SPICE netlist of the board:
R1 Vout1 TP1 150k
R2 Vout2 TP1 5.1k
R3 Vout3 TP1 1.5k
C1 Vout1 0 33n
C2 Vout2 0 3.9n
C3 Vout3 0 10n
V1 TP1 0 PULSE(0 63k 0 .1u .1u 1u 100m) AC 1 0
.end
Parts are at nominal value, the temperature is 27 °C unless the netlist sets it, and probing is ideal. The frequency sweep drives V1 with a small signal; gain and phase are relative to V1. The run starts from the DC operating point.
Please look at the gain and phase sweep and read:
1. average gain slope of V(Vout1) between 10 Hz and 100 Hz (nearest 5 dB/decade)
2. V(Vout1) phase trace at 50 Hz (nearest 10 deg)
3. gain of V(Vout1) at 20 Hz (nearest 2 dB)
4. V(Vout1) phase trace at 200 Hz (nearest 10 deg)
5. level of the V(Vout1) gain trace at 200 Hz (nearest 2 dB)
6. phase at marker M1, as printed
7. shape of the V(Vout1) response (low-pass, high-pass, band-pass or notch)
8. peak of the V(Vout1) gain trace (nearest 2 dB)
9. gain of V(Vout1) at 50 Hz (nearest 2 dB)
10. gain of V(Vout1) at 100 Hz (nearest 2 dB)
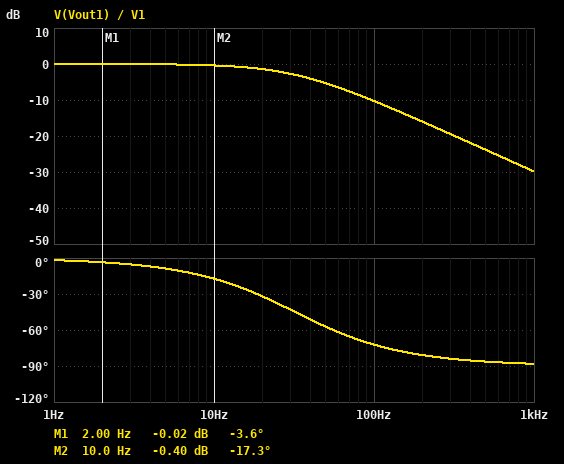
-10 dB/decade
-60 deg
-2 dB
-80 deg
-16 dB
-3.6 deg
low-pass
0 dB
-6 dB
-10 dB
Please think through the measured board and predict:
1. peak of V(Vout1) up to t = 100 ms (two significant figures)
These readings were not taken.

14 V
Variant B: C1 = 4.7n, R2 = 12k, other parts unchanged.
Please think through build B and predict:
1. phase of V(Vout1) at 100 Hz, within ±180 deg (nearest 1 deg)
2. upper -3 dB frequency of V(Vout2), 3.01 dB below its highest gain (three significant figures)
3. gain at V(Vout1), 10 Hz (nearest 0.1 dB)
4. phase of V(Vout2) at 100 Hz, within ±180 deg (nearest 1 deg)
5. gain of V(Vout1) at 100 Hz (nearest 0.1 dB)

-24 deg
3.40 kHz
0 dB
-2 deg
-0.8 dB
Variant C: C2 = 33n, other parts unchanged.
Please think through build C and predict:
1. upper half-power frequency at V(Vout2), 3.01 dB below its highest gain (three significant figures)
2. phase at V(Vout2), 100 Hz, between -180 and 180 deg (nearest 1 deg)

946 Hz
-6 deg
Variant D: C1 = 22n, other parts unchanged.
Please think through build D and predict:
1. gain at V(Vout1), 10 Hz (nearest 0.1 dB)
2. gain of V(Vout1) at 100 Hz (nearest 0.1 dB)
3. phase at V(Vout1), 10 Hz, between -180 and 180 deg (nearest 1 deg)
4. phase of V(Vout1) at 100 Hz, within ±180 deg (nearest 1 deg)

-0.2 dB
-7.2 dB
-12 deg
-64 deg
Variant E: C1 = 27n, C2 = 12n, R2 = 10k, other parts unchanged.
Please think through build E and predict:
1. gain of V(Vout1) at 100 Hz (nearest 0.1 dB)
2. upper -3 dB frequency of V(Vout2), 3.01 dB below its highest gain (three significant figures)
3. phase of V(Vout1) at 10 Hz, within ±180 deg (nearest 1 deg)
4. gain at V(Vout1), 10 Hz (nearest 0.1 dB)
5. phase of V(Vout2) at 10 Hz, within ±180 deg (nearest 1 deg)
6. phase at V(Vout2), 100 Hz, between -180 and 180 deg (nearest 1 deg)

-8.7 dB
1.33 kHz
-14 deg
-0.3 dB
0 deg
-4 deg
